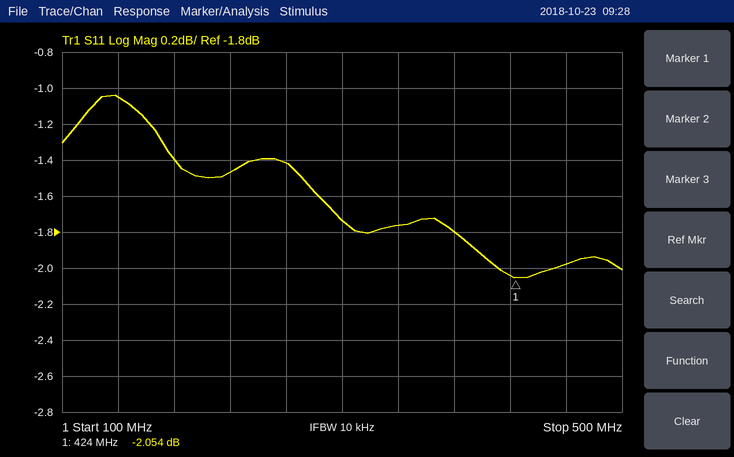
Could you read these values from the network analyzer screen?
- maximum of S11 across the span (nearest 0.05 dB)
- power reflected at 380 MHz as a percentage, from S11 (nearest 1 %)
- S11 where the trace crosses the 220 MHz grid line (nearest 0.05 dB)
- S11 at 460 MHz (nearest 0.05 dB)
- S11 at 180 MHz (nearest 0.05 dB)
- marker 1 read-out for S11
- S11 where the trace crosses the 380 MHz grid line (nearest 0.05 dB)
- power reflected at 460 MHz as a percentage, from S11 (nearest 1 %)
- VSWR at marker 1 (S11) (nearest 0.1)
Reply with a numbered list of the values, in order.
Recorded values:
1. -1.05 dB
2. 66 %
3. -1.45 dB
4. -2.00 dB
5. -1.40 dB
6. -2.054 dB
7. -1.80 dB
8. 63 %
9. 8.5
